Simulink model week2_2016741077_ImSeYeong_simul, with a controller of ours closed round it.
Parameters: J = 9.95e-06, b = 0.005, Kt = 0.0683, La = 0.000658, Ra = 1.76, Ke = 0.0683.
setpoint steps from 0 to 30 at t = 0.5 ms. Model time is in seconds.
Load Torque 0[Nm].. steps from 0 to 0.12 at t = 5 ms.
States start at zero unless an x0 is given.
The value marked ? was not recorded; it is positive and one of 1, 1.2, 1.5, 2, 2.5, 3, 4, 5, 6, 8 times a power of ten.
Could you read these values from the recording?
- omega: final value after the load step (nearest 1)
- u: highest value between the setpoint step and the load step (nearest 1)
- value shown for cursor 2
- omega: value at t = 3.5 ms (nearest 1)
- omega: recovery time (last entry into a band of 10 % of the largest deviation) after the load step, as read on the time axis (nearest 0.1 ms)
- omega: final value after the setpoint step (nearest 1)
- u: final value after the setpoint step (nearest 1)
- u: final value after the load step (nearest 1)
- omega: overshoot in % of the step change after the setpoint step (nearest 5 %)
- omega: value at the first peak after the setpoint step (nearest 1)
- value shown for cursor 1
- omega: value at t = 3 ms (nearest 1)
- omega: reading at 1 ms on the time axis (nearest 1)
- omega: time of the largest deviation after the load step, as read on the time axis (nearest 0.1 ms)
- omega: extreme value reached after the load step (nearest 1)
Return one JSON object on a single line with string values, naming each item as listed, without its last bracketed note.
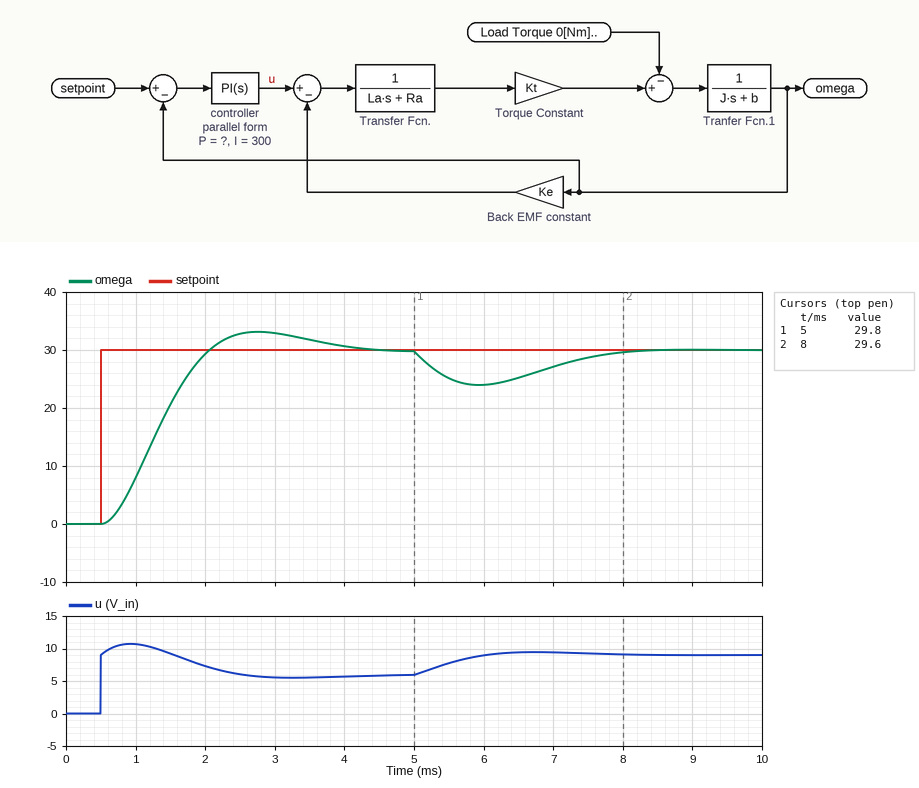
{"omega: final value after the load step": "30", "u: highest value between the setpoint step and the load step": "11", "value shown for cursor 2": "29.6", "omega: value at t = 3.5 ms": "32", "omega: recovery time (last entry into a band of 10 % of the largest deviation) after the load step, as read on the time axis": "7.9 ms", "omega: final value after the setpoint step": "30", "u: final value after the setpoint step": "6", "u: final value after the load step": "9", "omega: overshoot in % of the step change after the setpoint step": "10 %", "omega: value at the first peak after the setpoint step": "33", "value shown for cursor 1": "29.8", "omega: value at t = 3 ms": "33", "omega: reading at 1 ms on the time axis": "8", "omega: time of the largest deviation after the load step, as read on the time axis": "5.9 ms", "omega: extreme value reached after the load step": "24"}
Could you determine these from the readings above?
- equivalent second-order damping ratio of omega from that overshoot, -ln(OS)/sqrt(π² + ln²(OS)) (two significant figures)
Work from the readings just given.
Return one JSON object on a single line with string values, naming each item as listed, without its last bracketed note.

{"equivalent second-order damping ratio of omega from that overshoot, -ln(OS)/sqrt(π² + ln²(OS))": "0.59"}
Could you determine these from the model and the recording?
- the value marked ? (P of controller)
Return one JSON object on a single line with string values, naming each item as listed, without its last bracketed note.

{"the value marked ?": "0.3"}
